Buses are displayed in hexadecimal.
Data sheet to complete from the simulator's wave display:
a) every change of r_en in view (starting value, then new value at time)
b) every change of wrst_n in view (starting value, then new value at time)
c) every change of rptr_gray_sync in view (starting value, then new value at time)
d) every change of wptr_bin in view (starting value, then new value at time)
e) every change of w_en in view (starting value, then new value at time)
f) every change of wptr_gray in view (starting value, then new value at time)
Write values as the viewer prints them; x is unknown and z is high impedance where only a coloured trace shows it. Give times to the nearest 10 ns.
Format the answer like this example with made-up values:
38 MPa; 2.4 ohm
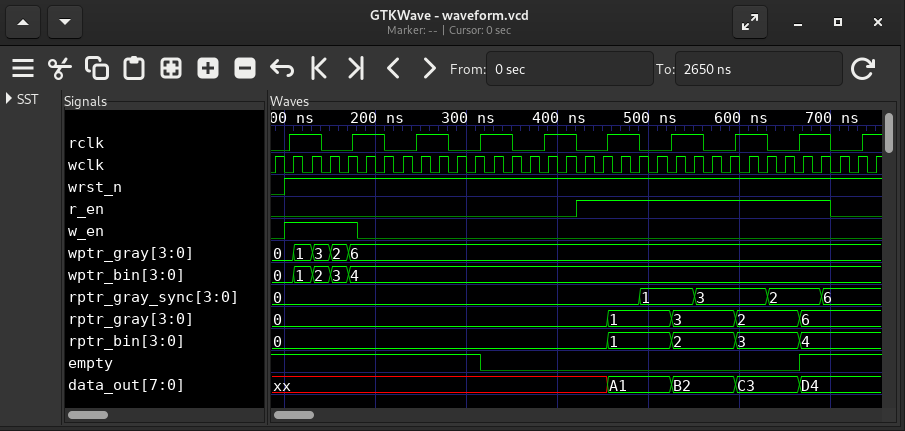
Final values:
0, 1 at 420 ns, 0 at 700 ns; 0, 1 at 100 ns; 0, 1 at 490 ns, 3 at 550 ns, 2 at 630 ns, 6 at 690 ns; 0, 1 at 110 ns, 2 at 130 ns, 3 at 150 ns, 4 at 170 ns; 0, 1 at 100 ns, 0 at 180 ns; 0, 1 at 110 ns, 3 at 130 ns, 2 at 150 ns, 6 at 170 ns
